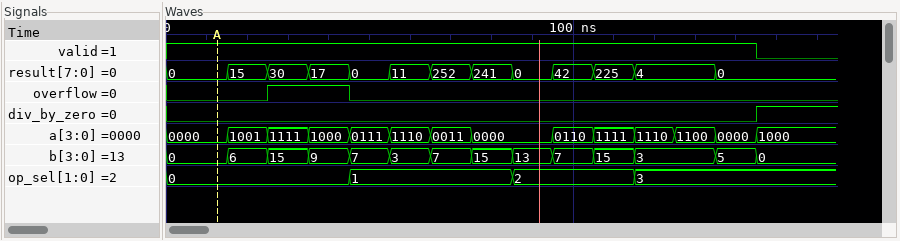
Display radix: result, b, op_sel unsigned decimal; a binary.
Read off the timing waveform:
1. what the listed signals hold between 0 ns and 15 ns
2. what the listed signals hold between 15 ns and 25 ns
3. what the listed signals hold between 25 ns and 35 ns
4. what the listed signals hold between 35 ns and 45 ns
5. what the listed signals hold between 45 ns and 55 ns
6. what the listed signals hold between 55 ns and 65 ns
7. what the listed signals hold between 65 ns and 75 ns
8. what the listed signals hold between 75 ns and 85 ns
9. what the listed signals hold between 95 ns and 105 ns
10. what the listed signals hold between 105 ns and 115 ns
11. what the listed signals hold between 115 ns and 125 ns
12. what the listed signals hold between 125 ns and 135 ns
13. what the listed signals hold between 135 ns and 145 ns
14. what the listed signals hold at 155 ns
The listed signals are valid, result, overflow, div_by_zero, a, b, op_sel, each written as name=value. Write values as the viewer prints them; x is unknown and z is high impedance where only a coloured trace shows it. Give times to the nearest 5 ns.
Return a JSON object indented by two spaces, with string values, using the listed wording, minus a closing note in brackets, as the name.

{
  "what the listed signals hold between 0 ns and 15 ns": "valid=1, result=0, overflow=0, div_by_zero=0, a=0000, b=0, op_sel=0",
  "what the listed signals hold between 15 ns and 25 ns": "valid=1, result=15, overflow=0, div_by_zero=0, a=1001, b=6, op_sel=0",
  "what the listed signals hold between 25 ns and 35 ns": "valid=1, result=30, overflow=1, div_by_zero=0, a=1111, b=15, op_sel=0",
  "what the listed signals hold between 35 ns and 45 ns": "valid=1, result=17, overflow=1, div_by_zero=0, a=1000, b=9, op_sel=0",
  "what the listed signals hold between 45 ns and 55 ns": "valid=1, result=0, overflow=0, div_by_zero=0, a=0111, b=7, op_sel=1",
  "what the listed signals hold between 55 ns and 65 ns": "valid=1, result=11, overflow=0, div_by_zero=0, a=1110, b=3, op_sel=1",
  "what the listed signals hold between 65 ns and 75 ns": "valid=1, result=252, overflow=0, div_by_zero=0, a=0011, b=7, op_sel=1",
  "what the listed signals hold between 75 ns and 85 ns": "valid=1, result=241, overflow=0, div_by_zero=0, a=0000, b=15, op_sel=1",
  "what the listed signals hold between 95 ns and 105 ns": "valid=1, result=42, overflow=0, div_by_zero=0, a=0110, b=7, op_sel=2",
  "what the listed signals hold between 105 ns and 115 ns": "valid=1, result=225, overflow=0, div_by_zero=0, a=1111, b=15, op_sel=2",
  "what the listed signals hold between 115 ns and 125 ns": "valid=1, result=4, overflow=0, div_by_zero=0, a=1110, b=3, op_sel=3",
  "what the listed signals hold between 125 ns and 135 ns": "valid=1, result=4, overflow=0, div_by_zero=0, a=1100, b=3, op_sel=3",
  "what the listed signals hold between 135 ns and 145 ns": "valid=1, result=0, overflow=0, div_by_zero=0, a=0000, b=5, op_sel=3",
  "what the listed signals hold at 155 ns": "valid=0, result=0, overflow=0, div_by_zero=1, a=1000, b=0, op_sel=3"
}
